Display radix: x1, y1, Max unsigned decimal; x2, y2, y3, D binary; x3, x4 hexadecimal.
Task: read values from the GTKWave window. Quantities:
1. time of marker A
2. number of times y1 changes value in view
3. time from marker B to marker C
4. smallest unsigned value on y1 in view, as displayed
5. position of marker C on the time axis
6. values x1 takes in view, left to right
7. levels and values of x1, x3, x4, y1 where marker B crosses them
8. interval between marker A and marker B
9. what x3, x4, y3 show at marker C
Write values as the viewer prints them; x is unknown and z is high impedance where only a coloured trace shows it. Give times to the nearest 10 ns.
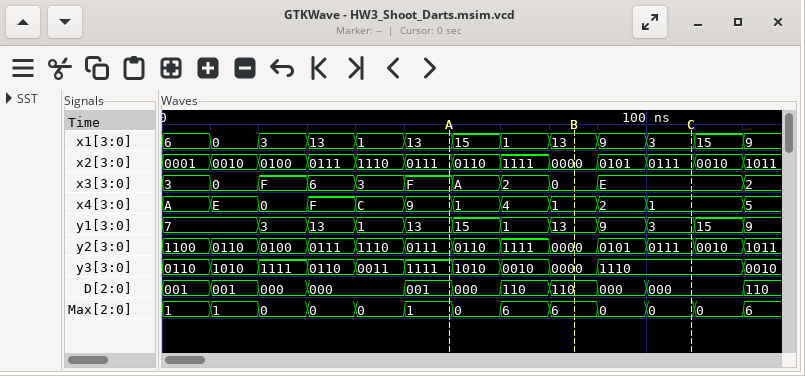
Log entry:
60 ns
11
20 ns
1
110 ns
6, 0, 3, 13, 1, 13, 15, 1, 13, 9, 3, 15, 9
x1=13, x3=0, x4=1, y1=13
30 ns
x3=E, x4=1, y3=1110
